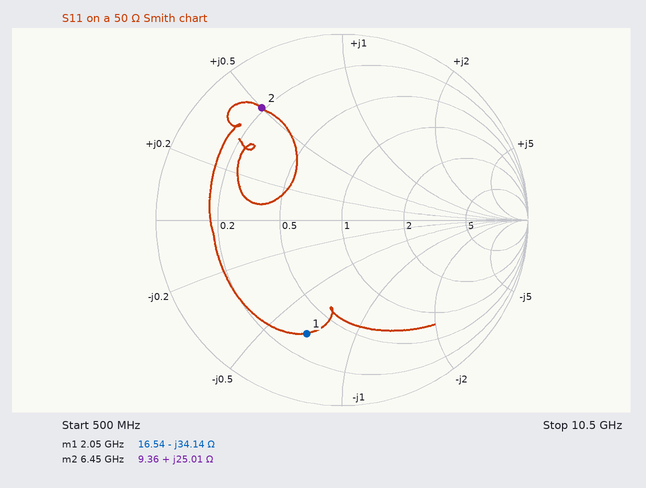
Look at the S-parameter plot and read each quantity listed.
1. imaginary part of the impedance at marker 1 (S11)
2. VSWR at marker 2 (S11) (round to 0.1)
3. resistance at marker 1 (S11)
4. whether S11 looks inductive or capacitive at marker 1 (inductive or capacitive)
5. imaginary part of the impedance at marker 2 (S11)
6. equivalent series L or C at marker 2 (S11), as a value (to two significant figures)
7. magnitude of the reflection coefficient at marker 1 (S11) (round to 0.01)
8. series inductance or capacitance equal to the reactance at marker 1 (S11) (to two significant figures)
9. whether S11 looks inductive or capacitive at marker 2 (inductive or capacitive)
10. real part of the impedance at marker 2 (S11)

-34.14 Ω
6.7
16.54 Ω
capacitive
+25.01 Ω
620 pH
0.64
2.3 pF
inductive
9.36 Ω
